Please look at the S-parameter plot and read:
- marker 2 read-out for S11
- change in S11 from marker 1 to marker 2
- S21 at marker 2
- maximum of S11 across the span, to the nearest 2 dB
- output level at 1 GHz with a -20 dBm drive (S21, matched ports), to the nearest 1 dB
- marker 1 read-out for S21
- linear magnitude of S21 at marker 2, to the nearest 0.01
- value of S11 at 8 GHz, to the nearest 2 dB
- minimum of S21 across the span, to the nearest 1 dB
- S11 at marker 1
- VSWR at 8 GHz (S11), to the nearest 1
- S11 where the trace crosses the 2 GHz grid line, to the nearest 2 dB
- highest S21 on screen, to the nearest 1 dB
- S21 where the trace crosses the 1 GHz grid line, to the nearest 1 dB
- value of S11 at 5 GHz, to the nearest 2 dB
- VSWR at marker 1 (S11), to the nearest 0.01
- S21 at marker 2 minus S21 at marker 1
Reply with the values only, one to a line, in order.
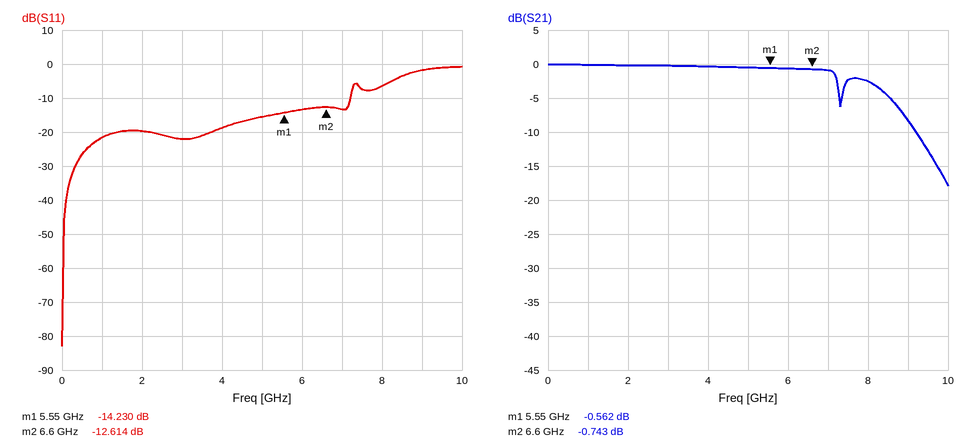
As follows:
-12.614 dB
1.616 dB
-0.743 dB
0 dB
-20 dBm
-0.562 dB
0.92
-6 dB
-18 dB
-14.230 dB
3
-20 dB
0 dB
0 dB
-16 dB
1.48
-0.181 dB
